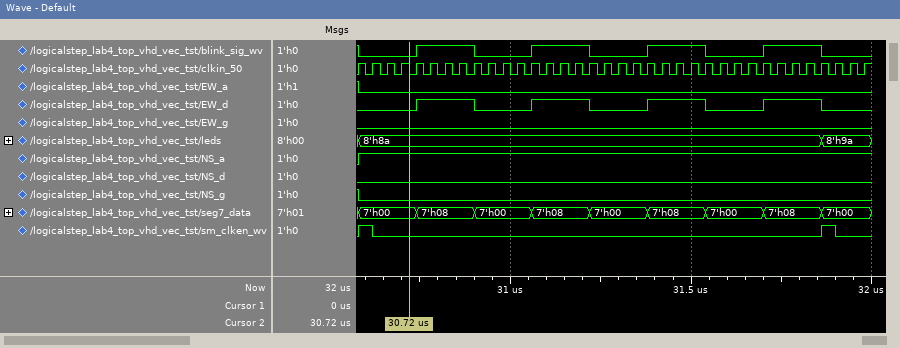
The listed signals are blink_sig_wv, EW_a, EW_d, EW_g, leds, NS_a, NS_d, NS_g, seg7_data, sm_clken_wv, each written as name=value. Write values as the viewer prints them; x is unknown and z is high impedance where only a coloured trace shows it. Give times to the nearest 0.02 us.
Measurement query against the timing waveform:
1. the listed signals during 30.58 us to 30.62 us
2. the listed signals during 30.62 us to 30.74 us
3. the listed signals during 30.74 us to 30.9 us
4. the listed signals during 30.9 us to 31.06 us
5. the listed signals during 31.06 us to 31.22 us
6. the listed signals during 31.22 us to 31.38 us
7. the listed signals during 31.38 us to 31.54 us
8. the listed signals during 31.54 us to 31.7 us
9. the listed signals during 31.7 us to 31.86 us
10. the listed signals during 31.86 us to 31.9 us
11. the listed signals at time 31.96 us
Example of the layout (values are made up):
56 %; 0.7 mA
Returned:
blink_sig_wv=0, EW_a=0, EW_d=0, EW_g=0, leds=8'h8a, NS_a=1, NS_d=0, NS_g=0, seg7_data=7'h00, sm_clken_wv=1; blink_sig_wv=0, EW_a=0, EW_d=0, EW_g=0, leds=8'h8a, NS_a=1, NS_d=0, NS_g=0, seg7_data=7'h00, sm_clken_wv=0; blink_sig_wv=1, EW_a=0, EW_d=1, EW_g=0, leds=8'h8a, NS_a=1, NS_d=0, NS_g=0, seg7_data=7'h08, sm_clken_wv=0; blink_sig_wv=0, EW_a=0, EW_d=0, EW_g=0, leds=8'h8a, NS_a=1, NS_d=0, NS_g=0, seg7_data=7'h00, sm_clken_wv=0; blink_sig_wv=1, EW_a=0, EW_d=1, EW_g=0, leds=8'h8a, NS_a=1, NS_d=0, NS_g=0, seg7_data=7'h08, sm_clken_wv=0; blink_sig_wv=0, EW_a=0, EW_d=0, EW_g=0, leds=8'h8a, NS_a=1, NS_d=0, NS_g=0, seg7_data=7'h00, sm_clken_wv=0; blink_sig_wv=1, EW_a=0, EW_d=1, EW_g=0, leds=8'h8a, NS_a=1, NS_d=0, NS_g=0, seg7_data=7'h08, sm_clken_wv=0; blink_sig_wv=0, EW_a=0, EW_d=0, EW_g=0, leds=8'h8a, NS_a=1, NS_d=0, NS_g=0, seg7_data=7'h00, sm_clken_wv=0; blink_sig_wv=1, EW_a=0, EW_d=1, EW_g=0, leds=8'h8a, NS_a=1, NS_d=0, NS_g=0, seg7_data=7'h08, sm_clken_wv=0; blink_sig_wv=0, EW_a=0, EW_d=0, EW_g=0, leds=8'h9a, NS_a=1, NS_d=0, NS_g=0, seg7_data=7'h00, sm_clken_wv=1; blink_sig_wv=0, EW_a=0, EW_d=0, EW_g=0, leds=8'h9a, NS_a=1, NS_d=0, NS_g=0, seg7_data=7'h00, sm_clken_wv=0
